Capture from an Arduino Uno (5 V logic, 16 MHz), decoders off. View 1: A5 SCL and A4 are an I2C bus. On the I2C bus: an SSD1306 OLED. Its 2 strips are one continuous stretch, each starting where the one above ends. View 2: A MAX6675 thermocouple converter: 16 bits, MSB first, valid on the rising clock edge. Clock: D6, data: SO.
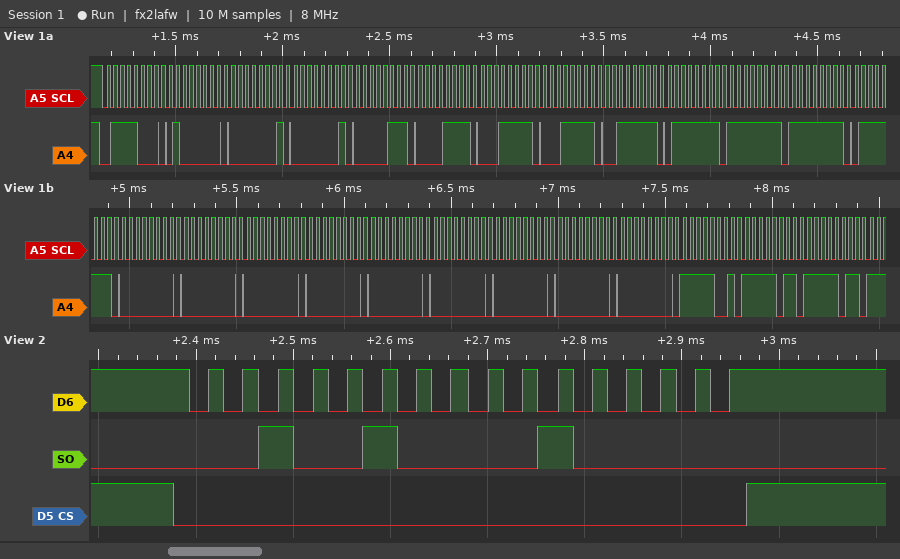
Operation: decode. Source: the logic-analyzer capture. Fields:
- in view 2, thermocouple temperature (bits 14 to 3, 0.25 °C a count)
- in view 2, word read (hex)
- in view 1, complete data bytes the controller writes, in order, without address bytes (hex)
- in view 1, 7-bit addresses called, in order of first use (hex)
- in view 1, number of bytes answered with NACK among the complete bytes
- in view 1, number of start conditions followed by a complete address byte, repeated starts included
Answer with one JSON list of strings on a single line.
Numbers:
["289.00 °C", "0x2420", "40 01 01 07 0F 1F 1F 3F 7F FF FF 7F 00 00 00 00 00 00 00 00 00 F9 FB FB", "0x3C", "0", "1"]
